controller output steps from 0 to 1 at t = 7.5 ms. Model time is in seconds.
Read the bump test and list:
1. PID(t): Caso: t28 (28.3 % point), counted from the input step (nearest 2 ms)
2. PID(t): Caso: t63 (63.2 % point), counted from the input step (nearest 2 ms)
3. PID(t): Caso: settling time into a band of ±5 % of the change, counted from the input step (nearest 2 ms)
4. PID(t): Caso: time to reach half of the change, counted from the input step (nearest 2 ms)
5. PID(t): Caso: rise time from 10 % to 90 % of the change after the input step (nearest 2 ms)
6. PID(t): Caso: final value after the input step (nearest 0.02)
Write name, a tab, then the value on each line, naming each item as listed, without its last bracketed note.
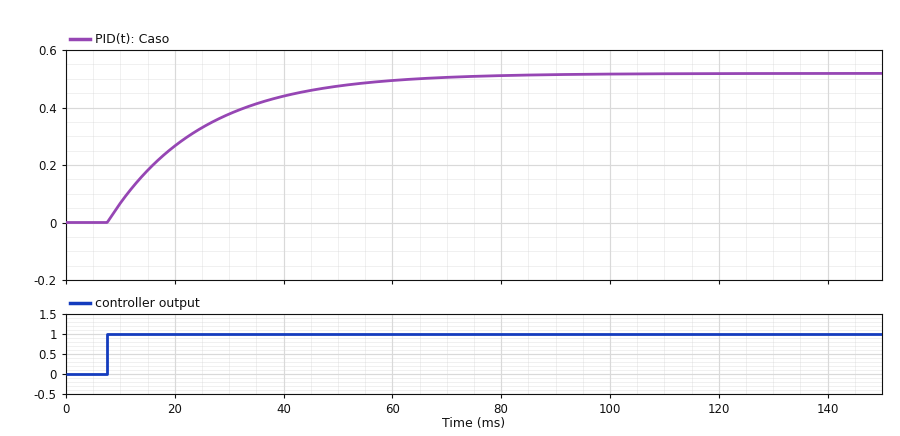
PID(t): Caso: t28 (28.3 % point), counted from the input step	6 ms
PID(t): Caso: t63 (63.2 % point), counted from the input step	18 ms
PID(t): Caso: settling time into a band of ±5 % of the change, counted from the input step	52 ms
PID(t): Caso: time to reach half of the change, counted from the input step	12 ms
PID(t): Caso: rise time from 10 % to 90 % of the change after the input step	38 ms
PID(t): Caso: final value after the input step	0.52
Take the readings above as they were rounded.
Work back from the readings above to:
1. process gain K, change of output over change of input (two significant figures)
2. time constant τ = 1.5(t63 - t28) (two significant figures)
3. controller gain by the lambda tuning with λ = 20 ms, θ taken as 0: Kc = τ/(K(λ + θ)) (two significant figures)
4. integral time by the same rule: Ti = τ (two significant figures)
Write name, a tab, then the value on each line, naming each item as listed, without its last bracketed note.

process gain K, change of output over change of input	0.52
time constant τ = 1.5(t63 - t28)	18 ms
controller gain by the lambda tuning with λ = 20 ms, θ taken as 0: Kc = τ/(K(λ + θ))	1.7
integral time by the same rule: Ti = τ	18 ms
